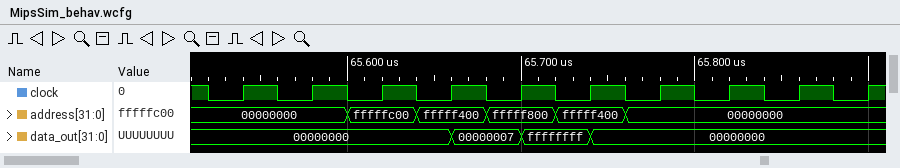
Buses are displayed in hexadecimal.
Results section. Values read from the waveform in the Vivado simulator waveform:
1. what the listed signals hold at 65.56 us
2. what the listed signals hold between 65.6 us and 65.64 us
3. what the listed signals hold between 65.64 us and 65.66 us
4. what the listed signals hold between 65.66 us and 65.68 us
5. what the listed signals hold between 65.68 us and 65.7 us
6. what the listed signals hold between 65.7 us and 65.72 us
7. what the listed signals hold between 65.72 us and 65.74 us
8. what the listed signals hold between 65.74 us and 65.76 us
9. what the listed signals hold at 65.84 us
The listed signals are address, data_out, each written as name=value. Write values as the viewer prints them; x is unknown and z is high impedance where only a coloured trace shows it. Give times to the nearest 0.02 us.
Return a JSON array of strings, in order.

["address=00000000, data_out=00000000", "address=fffffc00, data_out=00000000", "address=fffff400, data_out=00000000", "address=fffff400, data_out=00000007", "address=fffff800, data_out=00000007", "address=fffff800, data_out=ffffffff", "address=fffff400, data_out=ffffffff", "address=fffff400, data_out=00000000", "address=00000000, data_out=00000000"]
